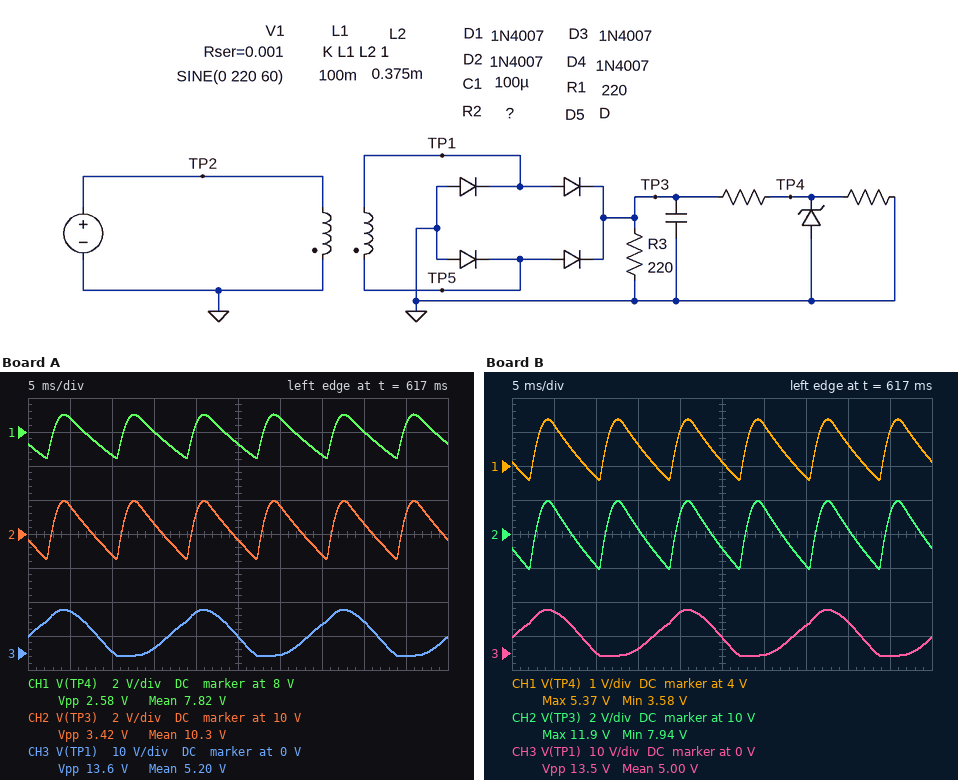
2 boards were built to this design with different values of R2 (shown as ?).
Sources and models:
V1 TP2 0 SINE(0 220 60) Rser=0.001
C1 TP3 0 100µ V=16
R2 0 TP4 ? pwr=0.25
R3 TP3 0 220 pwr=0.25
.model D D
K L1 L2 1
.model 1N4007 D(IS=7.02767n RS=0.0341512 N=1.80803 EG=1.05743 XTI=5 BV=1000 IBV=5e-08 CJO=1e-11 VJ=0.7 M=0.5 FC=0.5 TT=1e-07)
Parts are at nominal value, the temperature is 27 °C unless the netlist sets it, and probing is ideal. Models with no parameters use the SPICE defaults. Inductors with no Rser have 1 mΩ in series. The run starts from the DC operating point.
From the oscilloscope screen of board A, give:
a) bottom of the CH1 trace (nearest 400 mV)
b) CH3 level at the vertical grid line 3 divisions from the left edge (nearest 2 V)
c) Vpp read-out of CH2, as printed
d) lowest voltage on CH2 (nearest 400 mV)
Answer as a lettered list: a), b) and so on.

a) 6.4 V
b) 2 V
c) 3.42 V
d) 8.4 V
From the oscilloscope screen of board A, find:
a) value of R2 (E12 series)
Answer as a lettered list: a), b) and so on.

a) 680 Ω
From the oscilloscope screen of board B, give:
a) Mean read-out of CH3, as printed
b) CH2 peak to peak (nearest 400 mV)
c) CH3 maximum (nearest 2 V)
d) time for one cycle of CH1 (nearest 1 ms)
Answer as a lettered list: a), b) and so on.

a) 5.00 V
b) 4.0 V
c) 12 V
d) 8 ms
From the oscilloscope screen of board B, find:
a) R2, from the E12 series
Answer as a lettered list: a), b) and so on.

a) 180 Ω
